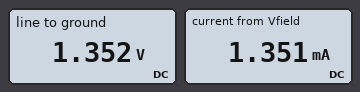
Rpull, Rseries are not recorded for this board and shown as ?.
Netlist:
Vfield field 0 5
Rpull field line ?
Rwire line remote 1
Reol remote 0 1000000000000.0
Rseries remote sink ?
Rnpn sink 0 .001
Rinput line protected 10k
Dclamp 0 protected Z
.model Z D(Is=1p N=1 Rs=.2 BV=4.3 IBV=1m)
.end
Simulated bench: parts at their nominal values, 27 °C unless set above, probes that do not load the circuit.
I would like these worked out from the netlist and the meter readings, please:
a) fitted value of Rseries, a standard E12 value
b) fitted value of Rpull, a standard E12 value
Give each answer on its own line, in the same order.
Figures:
1 kΩ
2.7 kΩ
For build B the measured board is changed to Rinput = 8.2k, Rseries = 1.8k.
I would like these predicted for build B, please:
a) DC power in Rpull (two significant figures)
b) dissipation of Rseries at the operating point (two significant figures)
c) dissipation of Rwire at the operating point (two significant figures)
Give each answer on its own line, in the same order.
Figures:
3.3 mW
2.2 mW
1.2 µW
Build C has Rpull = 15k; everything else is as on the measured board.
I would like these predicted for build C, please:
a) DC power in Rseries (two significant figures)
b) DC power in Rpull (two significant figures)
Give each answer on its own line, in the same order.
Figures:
98 µW
1.5 mW
